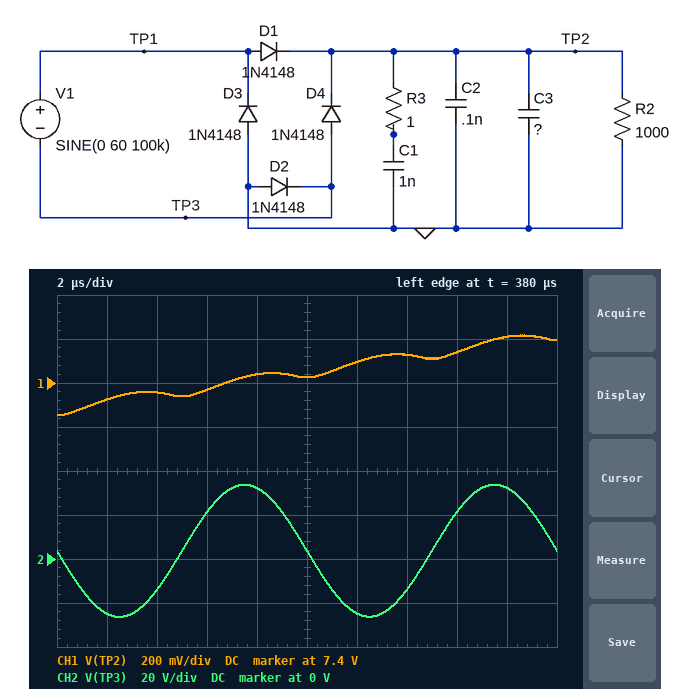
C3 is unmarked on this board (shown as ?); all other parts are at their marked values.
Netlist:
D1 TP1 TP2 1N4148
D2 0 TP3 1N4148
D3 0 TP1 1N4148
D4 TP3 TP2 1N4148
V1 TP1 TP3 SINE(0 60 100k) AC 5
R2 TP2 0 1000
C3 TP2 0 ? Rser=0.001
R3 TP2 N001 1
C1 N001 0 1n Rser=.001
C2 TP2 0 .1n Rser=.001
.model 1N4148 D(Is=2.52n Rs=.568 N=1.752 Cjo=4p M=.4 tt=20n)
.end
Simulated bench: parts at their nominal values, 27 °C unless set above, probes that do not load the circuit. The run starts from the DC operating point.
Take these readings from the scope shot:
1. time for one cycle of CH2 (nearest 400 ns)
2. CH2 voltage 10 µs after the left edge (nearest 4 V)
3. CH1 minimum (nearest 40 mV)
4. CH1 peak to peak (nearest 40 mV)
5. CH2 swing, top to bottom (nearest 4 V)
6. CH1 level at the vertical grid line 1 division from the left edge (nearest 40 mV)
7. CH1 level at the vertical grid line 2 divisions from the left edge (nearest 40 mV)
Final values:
10.0 µs
4 V
7.24 V
360 mV
60 V
7.32 V
7.36 V
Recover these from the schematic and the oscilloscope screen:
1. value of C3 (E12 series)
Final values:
1.5 mF
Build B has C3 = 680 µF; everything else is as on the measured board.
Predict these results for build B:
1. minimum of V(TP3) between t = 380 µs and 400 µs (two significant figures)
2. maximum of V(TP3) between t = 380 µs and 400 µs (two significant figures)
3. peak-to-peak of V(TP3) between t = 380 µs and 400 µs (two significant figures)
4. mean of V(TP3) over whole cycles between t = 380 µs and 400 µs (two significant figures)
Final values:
-23 V
37 V
60 V
7.3 V
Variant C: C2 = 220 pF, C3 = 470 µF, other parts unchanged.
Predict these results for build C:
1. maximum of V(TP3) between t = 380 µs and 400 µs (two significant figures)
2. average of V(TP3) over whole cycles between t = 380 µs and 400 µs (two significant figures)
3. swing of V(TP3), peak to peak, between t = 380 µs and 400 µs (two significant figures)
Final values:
40 V
9.7 V
60 V
